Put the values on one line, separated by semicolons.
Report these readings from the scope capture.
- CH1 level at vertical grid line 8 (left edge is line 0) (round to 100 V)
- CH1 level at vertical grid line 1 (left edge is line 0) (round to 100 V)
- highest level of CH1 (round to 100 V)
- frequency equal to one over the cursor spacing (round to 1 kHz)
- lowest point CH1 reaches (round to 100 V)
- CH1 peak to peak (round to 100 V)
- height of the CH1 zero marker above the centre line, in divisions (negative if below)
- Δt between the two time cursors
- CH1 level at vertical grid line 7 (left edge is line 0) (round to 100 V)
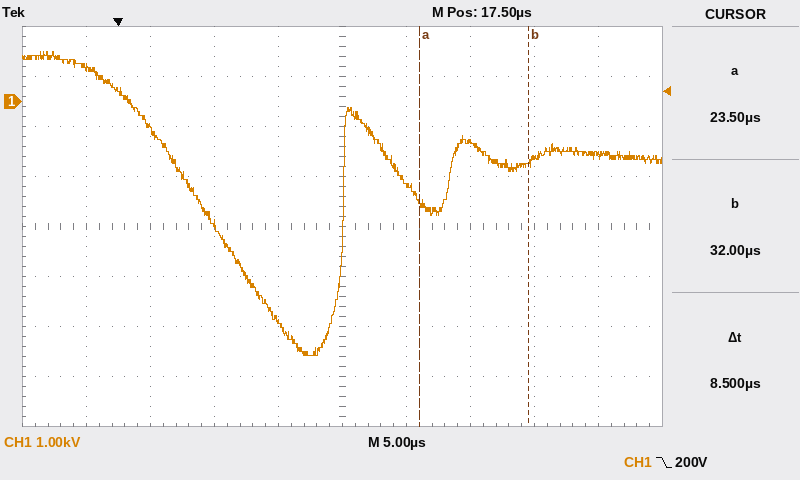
-1.1 kV; 700 V; 1.0 kV; 118 kHz; -5.1 kV; 6.1 kV; +2.5 div; 8.5 µs; -800 V
